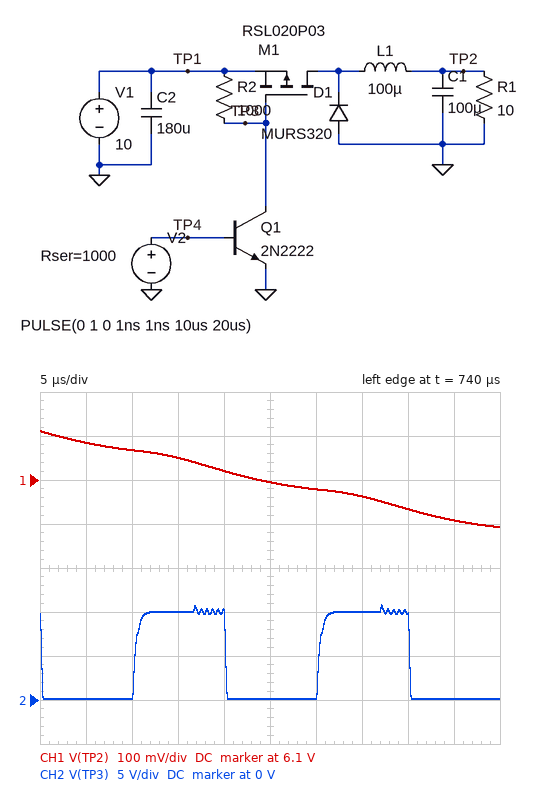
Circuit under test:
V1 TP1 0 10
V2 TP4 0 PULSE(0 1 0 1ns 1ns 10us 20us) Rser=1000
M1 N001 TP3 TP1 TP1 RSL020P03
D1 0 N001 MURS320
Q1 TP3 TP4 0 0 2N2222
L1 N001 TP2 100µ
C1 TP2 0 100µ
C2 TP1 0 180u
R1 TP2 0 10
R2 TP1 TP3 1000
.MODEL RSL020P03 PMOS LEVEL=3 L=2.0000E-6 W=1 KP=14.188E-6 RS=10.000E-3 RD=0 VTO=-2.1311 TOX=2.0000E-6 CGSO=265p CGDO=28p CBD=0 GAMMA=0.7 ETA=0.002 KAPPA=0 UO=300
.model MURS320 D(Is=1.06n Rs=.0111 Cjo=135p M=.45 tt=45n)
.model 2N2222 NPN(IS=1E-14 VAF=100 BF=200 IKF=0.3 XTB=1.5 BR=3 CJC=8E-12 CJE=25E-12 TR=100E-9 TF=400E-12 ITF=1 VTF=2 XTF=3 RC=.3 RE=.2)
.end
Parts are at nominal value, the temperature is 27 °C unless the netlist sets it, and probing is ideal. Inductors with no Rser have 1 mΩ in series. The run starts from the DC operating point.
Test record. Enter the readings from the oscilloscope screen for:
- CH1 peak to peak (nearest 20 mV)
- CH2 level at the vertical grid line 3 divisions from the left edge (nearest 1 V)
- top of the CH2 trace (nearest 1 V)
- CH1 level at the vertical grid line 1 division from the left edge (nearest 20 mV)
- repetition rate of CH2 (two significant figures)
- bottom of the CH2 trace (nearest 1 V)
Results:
220 mV
10 V
11 V
6.18 V
50 kHz
0 V
